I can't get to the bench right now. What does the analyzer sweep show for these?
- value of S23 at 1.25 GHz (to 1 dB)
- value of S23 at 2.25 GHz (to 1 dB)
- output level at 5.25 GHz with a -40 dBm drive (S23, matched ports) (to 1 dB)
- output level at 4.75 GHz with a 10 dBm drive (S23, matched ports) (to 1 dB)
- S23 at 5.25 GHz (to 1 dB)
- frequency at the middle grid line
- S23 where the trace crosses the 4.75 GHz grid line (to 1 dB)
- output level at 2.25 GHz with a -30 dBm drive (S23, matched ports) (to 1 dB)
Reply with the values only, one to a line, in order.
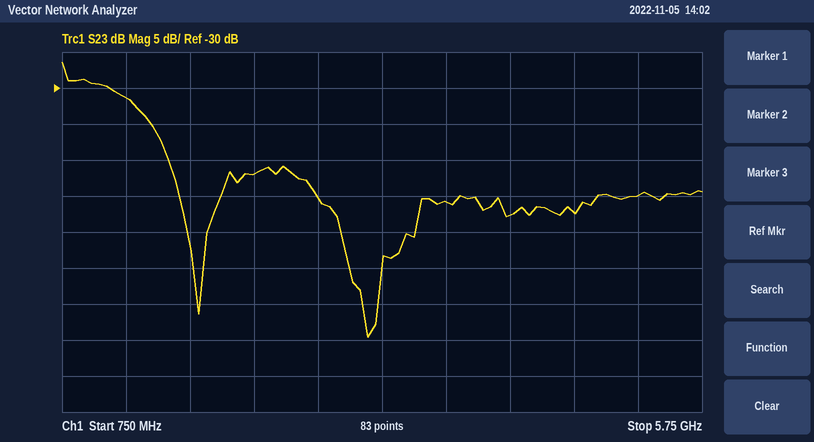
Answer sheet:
-31 dB
-42 dB
-85 dBm
-37 dBm
-45 dB
3.25 GHz
-47 dB
-72 dBm
